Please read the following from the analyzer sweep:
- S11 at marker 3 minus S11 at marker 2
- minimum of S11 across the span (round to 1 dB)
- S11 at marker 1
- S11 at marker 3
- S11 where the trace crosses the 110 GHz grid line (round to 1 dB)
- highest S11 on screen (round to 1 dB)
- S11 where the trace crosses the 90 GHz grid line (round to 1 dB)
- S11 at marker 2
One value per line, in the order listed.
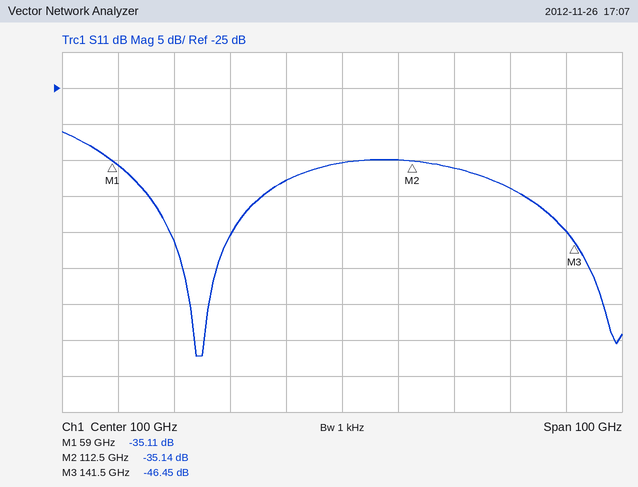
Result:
-11.31 dB
-62 dB
-35.11 dB
-46.45 dB
-35 dB
-31 dB
-38 dB
-35.14 dB
